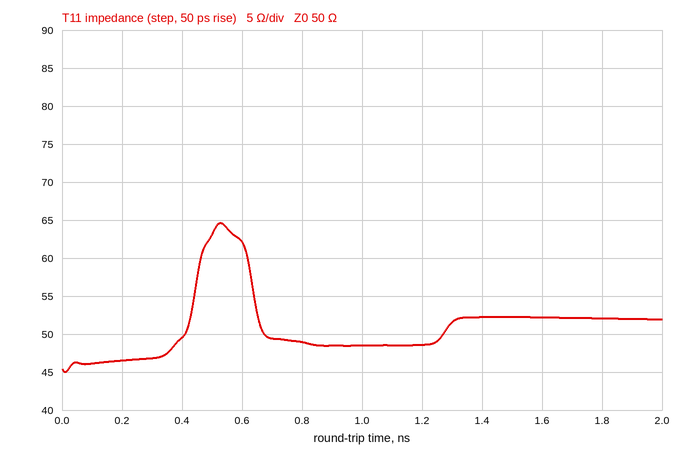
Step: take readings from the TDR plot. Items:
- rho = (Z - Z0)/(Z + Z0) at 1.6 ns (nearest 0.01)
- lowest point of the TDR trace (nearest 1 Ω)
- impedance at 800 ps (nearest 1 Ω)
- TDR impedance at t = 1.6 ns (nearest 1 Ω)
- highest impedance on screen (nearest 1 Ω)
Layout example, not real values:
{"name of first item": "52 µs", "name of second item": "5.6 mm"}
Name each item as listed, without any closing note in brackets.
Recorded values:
{"rho = (Z - Z0)/(Z + Z0) at 1.6 ns": "+0.02", "lowest point of the TDR trace": "45 Ω", "impedance at 800 ps": "49 Ω", "TDR impedance at t = 1.6 ns": "52 Ω", "highest impedance on screen": "65 Ω"}
